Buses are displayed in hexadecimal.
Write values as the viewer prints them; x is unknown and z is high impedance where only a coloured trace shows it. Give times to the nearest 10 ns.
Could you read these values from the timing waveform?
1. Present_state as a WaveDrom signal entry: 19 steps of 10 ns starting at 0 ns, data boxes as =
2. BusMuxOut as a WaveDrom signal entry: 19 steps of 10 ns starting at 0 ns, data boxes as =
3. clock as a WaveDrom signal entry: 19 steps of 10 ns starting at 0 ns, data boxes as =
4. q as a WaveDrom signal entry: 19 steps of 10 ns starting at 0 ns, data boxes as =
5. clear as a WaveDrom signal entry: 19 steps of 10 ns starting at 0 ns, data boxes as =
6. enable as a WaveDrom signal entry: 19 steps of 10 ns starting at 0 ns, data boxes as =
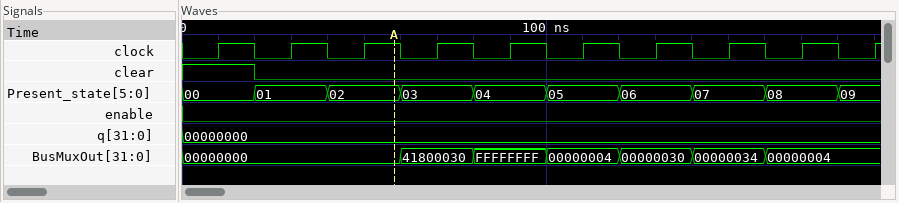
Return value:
{name: 'Present_state', wave: '=.=.=.=.=.=.=.=.=.=', data: '00 01 02 03 04 05 06 07 08 09'}
{name: 'BusMuxOut', wave: '=.....=.=.=.=.=.=..', data: '00000000 41800030 FFFFFFFF 00000004 00000030 00000034 00000004'}
{name: 'clock', wave: '0101010101010101010'}
{name: 'q', wave: '=..................', data: '00000000'}
{name: 'clear', wave: '1.0................'}
{name: 'enable', wave: '0..................'}
